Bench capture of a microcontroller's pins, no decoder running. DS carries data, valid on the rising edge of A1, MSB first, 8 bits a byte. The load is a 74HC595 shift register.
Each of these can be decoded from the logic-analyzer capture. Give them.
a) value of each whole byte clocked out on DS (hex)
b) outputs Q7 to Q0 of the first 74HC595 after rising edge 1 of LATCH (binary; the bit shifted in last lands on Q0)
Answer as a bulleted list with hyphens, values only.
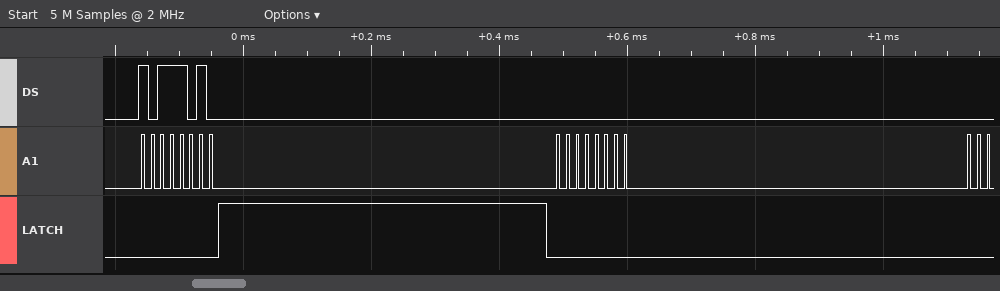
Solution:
- BA 00
- 10111010
